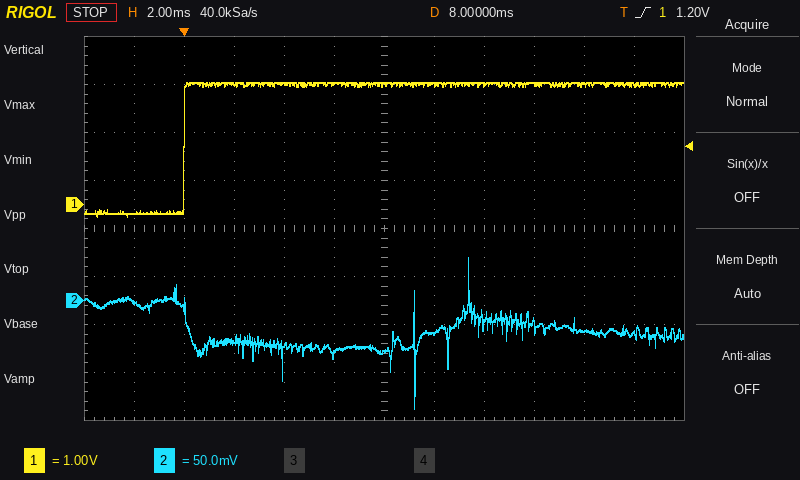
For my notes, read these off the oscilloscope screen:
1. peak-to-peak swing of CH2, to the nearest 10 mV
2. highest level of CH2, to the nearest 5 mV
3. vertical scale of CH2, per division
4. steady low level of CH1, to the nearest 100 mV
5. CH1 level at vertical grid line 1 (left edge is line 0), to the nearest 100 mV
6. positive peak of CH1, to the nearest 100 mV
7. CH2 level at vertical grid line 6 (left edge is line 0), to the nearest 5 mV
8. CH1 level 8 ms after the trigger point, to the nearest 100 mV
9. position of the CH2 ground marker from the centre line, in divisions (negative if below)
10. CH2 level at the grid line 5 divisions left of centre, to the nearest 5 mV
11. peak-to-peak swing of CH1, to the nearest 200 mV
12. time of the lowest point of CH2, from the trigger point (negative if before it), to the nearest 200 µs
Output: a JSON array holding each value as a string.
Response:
["160 mV", "45 mV", "50 mV", "-200 mV", "-200 mV", "2.5 V", "-55 mV", "2.5 V", "-1.5 div", "0 mV", "2.8 V", "+9.2 ms"]
